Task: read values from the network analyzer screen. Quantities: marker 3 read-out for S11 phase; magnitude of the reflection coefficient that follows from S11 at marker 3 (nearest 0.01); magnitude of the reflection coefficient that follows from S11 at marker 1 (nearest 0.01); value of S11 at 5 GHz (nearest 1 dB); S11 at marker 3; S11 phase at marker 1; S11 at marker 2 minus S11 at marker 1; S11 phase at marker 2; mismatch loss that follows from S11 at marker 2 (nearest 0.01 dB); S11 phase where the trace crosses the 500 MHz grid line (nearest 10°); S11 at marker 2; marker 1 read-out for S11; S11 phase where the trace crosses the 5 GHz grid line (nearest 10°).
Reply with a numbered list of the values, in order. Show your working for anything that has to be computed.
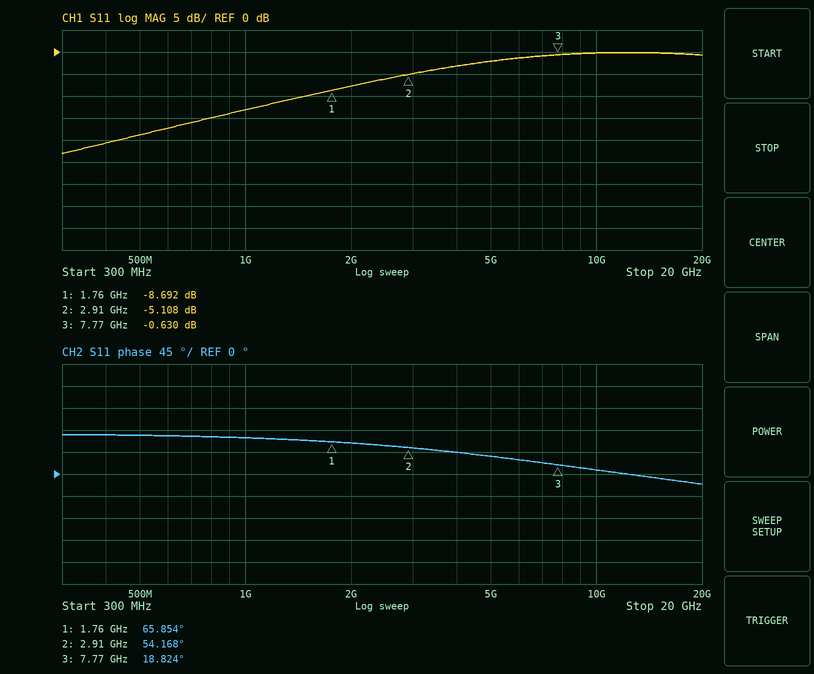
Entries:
1. 18.824°
2. 10^(-0.63/20) ≈ 0.93
3. 10^(-8.692/20) ≈ 0.37
4. -2 dB
5. -0.630 dB
6. 65.854°
7. -5.108 − (-8.692) = 3.584 dB
8. 54.168°
9. −10 log10(1 − 10^(-5.108/10)) ≈ 1.60 dB
10. 80°
11. -5.108 dB
12. -8.692 dB
13. 40°
